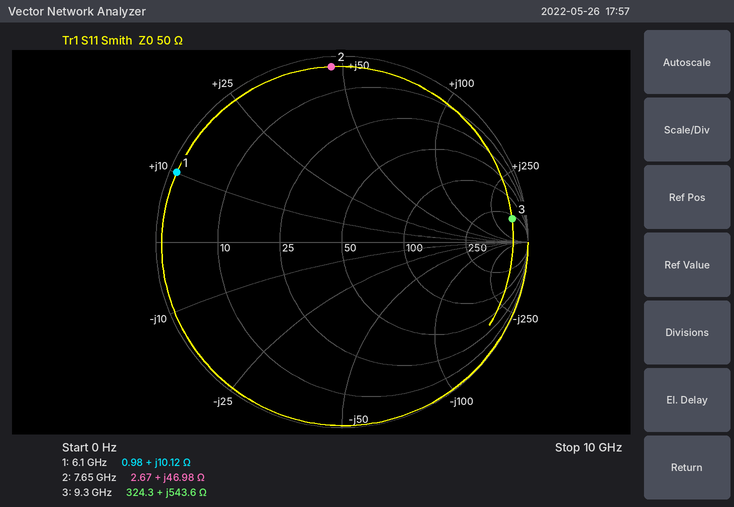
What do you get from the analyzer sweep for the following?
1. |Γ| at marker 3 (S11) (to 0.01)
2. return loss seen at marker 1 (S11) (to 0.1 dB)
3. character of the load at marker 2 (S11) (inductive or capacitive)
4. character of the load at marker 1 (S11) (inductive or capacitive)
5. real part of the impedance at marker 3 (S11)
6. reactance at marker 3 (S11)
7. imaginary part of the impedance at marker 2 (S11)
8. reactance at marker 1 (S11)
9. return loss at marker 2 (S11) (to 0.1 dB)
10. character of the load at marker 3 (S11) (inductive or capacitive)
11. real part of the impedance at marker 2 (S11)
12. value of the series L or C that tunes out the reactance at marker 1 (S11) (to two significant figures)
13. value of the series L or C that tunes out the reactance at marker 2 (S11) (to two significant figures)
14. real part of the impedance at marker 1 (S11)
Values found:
0.92
0.3 dB
inductive
inductive
324.3 Ω
+543.6 Ω
+46.98 Ω
+10.12 Ω
0.5 dB
inductive
2.67 Ω
2.6 pF
440 fF
0.98 Ω
